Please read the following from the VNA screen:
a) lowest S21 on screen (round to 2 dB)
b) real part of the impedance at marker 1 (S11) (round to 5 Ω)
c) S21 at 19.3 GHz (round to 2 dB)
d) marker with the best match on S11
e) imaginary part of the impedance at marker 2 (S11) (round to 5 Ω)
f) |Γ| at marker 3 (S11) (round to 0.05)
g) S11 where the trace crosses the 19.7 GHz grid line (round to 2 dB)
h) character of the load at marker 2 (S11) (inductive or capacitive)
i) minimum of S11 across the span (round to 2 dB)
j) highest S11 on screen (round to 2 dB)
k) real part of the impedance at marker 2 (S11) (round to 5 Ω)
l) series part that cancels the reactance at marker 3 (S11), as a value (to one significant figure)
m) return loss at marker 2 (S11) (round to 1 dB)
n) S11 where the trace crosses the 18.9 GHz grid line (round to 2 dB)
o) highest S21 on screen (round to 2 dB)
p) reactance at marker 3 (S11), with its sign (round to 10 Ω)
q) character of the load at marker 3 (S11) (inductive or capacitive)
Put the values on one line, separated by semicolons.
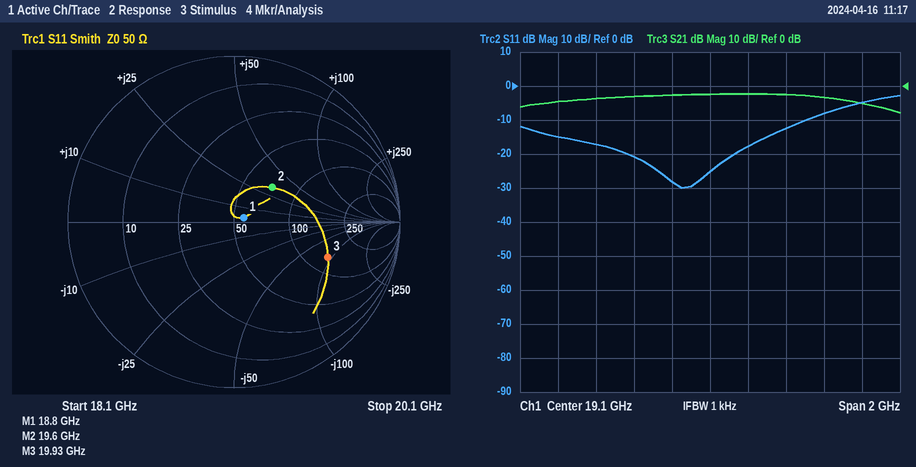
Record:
-8 dB; 55 Ω; -2 dB; marker 1; +35 Ω; 0.60; -8 dB; inductive; -30 dB; -2 dB; 70 Ω; 700 pH; 10 dB; -28 dB; -2 dB; -90 Ω; capacitive
